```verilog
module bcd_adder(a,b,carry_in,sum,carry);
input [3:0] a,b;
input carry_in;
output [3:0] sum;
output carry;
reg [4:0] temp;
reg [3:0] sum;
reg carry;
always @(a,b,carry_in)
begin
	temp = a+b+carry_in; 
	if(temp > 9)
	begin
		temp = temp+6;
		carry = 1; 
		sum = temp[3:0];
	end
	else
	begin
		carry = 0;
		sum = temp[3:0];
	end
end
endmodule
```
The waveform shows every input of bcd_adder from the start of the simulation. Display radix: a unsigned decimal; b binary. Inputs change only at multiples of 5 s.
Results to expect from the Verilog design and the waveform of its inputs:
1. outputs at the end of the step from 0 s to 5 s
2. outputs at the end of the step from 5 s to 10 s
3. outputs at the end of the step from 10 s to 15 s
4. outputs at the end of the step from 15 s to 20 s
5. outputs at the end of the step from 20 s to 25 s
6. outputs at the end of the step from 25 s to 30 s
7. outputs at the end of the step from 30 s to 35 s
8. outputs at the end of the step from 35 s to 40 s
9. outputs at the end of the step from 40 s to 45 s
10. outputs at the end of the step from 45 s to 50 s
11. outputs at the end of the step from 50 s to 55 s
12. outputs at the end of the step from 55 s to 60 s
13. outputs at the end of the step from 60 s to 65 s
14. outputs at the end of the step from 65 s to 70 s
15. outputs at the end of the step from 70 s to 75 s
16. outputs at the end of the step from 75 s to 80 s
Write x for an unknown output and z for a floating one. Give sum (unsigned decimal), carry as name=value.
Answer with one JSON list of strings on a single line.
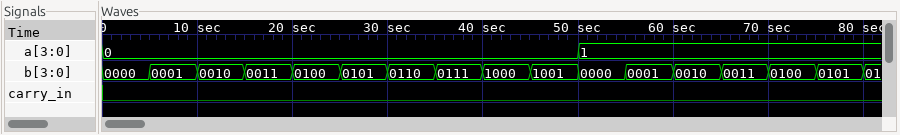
["sum=0, carry=0", "sum=1, carry=0", "sum=2, carry=0", "sum=3, carry=0", "sum=4, carry=0", "sum=5, carry=0", "sum=6, carry=0", "sum=7, carry=0", "sum=8, carry=0", "sum=9, carry=0", "sum=1, carry=0", "sum=2, carry=0", "sum=3, carry=0", "sum=4, carry=0", "sum=5, carry=0", "sum=6, carry=0"]
